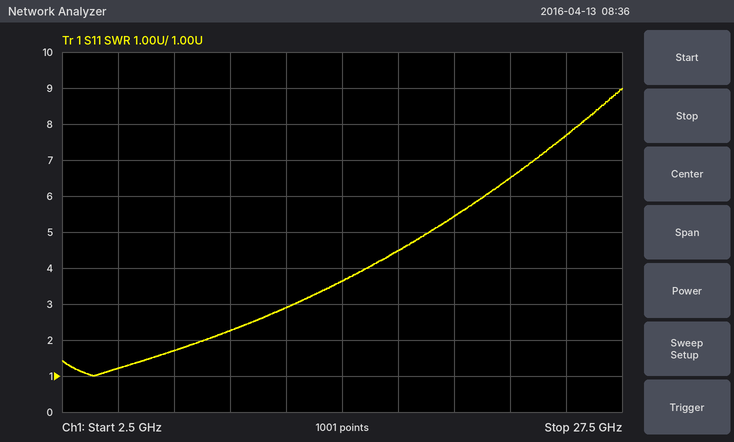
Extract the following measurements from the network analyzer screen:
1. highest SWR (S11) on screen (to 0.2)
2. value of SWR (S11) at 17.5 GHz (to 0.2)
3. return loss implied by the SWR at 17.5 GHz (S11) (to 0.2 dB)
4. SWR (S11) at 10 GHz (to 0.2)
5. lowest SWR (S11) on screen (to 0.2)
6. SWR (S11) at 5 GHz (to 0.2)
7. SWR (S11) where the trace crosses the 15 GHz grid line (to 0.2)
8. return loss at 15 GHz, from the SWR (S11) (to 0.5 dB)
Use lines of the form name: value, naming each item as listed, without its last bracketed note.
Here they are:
highest SWR (S11) on screen: 9.0
value of SWR (S11) at 17.5 GHz: 4.4
return loss implied by the SWR at 17.5 GHz (S11): 4.0 dB
SWR (S11) at 10 GHz: 2.2
lowest SWR (S11) on screen: 1.0
SWR (S11) at 5 GHz: 1.2
SWR (S11) where the trace crosses the 15 GHz grid line: 3.6
return loss at 15 GHz, from the SWR (S11): 5.0 dB
